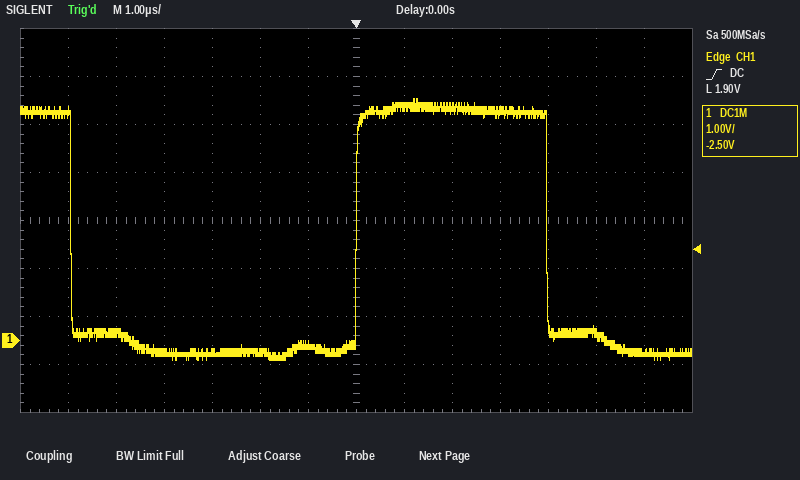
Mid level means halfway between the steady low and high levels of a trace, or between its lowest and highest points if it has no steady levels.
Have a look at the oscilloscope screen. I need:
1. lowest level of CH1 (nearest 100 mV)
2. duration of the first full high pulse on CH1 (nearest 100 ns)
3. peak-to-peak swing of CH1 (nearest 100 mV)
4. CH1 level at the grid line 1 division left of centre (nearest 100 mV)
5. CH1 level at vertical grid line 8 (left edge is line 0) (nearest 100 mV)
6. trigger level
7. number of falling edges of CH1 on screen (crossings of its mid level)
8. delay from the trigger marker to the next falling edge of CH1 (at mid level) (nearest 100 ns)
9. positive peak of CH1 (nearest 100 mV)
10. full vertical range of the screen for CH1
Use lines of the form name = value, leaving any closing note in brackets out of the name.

lowest level of CH1 = -400 mV
duration of the first full high pulse on CH1 = 4.0 µs
peak-to-peak swing of CH1 = 5.4 V
CH1 level at the grid line 1 division left of centre = -100 mV
CH1 level at vertical grid line 8 (left edge is line 0) = 4.9 V
trigger level = 1.90 V
number of falling edges of CH1 on screen = 2
delay from the trigger marker to the next falling edge of CH1 (at mid level) = 4.0 µs
positive peak of CH1 = 5.0 V
full vertical range of the screen for CH1 = 8 V
